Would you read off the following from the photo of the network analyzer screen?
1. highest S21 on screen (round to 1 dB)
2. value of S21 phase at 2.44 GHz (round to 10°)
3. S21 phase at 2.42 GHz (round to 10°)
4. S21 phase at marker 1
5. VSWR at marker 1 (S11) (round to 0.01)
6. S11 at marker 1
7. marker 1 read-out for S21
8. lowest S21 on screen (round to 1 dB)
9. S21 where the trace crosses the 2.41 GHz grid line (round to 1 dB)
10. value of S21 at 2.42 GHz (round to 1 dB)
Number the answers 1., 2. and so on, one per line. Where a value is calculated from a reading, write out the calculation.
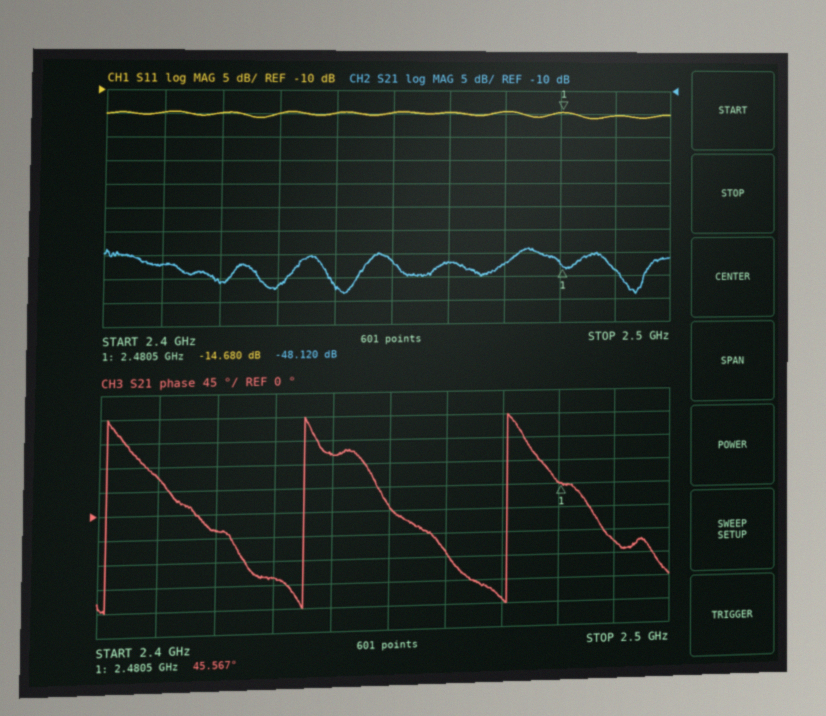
1. -44 dB
2. 110°
3. -30°
4. 45.567°
5. (1 + 0.1845)/(1 − 0.1845) ≈ 1.45
6. -14.680 dB
7. -48.120 dB
8. -54 dB
9. -47 dB
10. -51 dB
